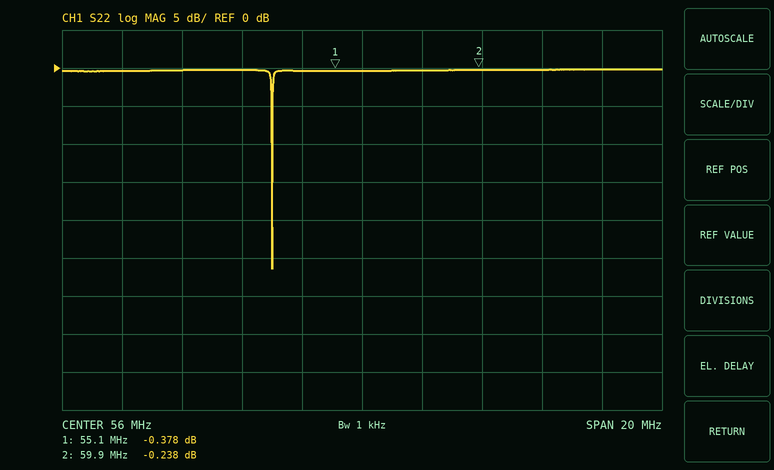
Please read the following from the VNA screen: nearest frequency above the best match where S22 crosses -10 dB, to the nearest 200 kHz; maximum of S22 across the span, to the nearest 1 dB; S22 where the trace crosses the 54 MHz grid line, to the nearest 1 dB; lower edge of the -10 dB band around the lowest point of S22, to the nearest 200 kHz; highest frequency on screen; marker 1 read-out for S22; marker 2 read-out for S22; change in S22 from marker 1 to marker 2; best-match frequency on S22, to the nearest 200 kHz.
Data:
53.0 MHz
0 dB
0 dB
53.0 MHz
66 MHz
-0.378 dB
-0.238 dB
0.140 dB
53.0 MHz
